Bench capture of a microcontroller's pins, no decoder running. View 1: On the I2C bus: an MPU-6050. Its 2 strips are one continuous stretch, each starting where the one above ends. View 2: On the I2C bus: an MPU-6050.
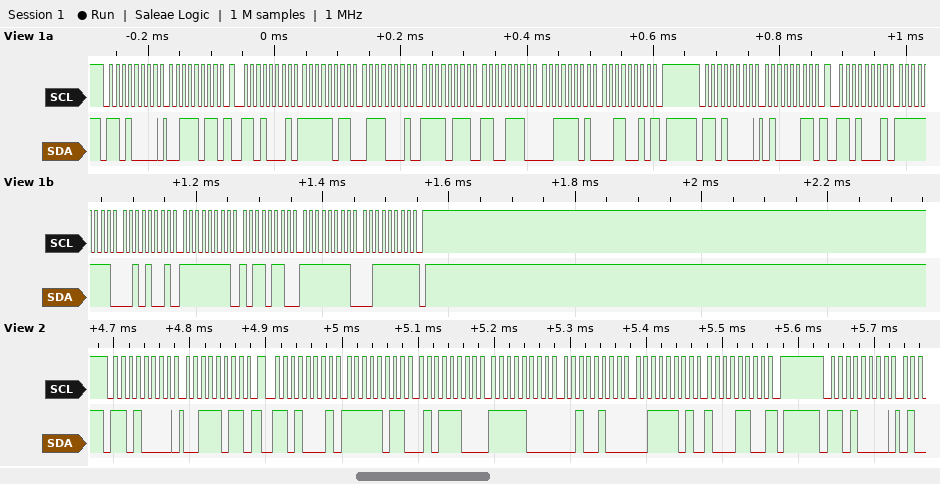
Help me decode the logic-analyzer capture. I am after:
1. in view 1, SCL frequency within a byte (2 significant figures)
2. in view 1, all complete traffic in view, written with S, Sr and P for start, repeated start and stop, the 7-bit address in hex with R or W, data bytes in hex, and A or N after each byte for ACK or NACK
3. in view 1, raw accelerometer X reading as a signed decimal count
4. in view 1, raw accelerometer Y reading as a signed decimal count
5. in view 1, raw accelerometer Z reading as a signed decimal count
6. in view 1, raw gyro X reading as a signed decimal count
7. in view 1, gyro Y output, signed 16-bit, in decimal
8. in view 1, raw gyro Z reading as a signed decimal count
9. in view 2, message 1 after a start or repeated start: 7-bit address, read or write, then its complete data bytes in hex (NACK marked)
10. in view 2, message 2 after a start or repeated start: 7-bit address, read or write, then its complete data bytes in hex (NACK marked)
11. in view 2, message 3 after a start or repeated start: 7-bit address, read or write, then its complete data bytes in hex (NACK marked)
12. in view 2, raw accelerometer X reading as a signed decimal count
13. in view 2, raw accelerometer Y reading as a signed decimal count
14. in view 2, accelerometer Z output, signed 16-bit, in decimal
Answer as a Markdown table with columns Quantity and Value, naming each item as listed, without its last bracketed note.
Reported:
| Quantity | Value |
|---|---|
| in view 1, SCL frequency within a byte | 100 kHz |
| in view 1, all complete traffic in view, written with S, Sr and P for start, repeated start and stop, the 7-bit address in hex with R or W, data bytes in hex, and A or N after each byte for ACK or NACK | S 68W A 3B A Sr 68R A FB A 71 A F7 A CE A 3D A 32 N P S 68W A 43 A Sr 68R A FF A 29 A FF A B6 A FF A 3F N P |
| in view 1, raw accelerometer X reading as a signed decimal count | -1167 |
| in view 1, raw accelerometer Y reading as a signed decimal count | -2098 |
| in view 1, raw accelerometer Z reading as a signed decimal count | 15666 |
| in view 1, raw gyro X reading as a signed decimal count | -215 |
| in view 1, gyro Y output, signed 16-bit, in decimal | -74 |
| in view 1, raw gyro Z reading as a signed decimal count | -193 |
| in view 2, message 1 after a start or repeated start: 7-bit address, read or write, then its complete data bytes in hex | 0x68 write: 3B |
| in view 2, message 2 after a start or repeated start: 7-bit address, read or write, then its complete data bytes in hex | 0x68 read: FB 5C F8 24 3D 8C NACK |
| in view 2, message 3 after a start or repeated start: 7-bit address, read or write, then its complete data bytes in hex | 0x68 write |
| in view 2, raw accelerometer X reading as a signed decimal count | -1188 |
| in view 2, raw accelerometer Y reading as a signed decimal count | -2012 |
| in view 2, accelerometer Z output, signed 16-bit, in decimal | 15756 |
